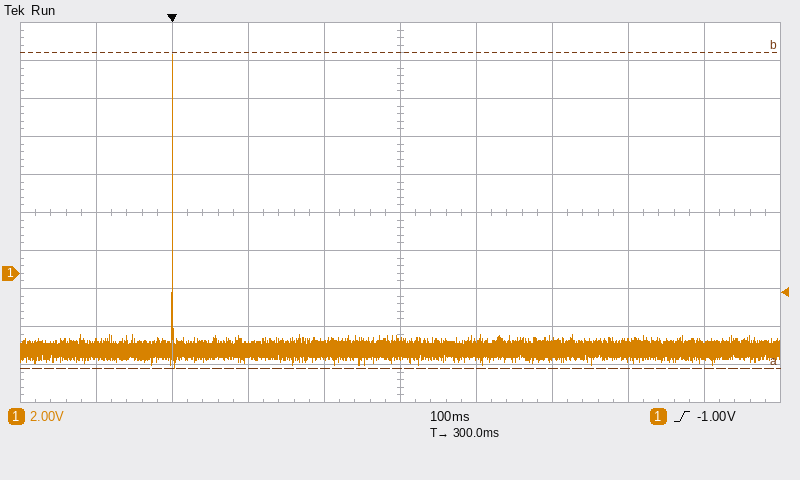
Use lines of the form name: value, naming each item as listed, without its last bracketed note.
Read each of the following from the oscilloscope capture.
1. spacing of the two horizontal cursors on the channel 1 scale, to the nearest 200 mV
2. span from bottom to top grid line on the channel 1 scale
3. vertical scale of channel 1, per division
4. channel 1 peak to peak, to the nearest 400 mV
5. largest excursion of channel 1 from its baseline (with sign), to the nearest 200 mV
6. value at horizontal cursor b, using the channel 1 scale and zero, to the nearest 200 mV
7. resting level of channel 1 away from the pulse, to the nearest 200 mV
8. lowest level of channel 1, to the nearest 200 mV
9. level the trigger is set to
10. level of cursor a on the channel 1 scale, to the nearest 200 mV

spacing of the two horizontal cursors on the channel 1 scale, to the nearest 200 mV: 16.6 V
span from bottom to top grid line on the channel 1 scale: 20 V
vertical scale of channel 1, per division: 2 V
channel 1 peak to peak, to the nearest 400 mV: 16.4 V
largest excursion of channel 1 from its baseline (with sign), to the nearest 200 mV: +15.6 V
value at horizontal cursor b, using the channel 1 scale and zero, to the nearest 200 mV: 11.6 V
resting level of channel 1 away from the pulse, to the nearest 200 mV: -4.0 V
lowest level of channel 1, to the nearest 200 mV: -5.0 V
level the trigger is set to: -1.00 V
level of cursor a on the channel 1 scale, to the nearest 200 mV: -5.0 V
